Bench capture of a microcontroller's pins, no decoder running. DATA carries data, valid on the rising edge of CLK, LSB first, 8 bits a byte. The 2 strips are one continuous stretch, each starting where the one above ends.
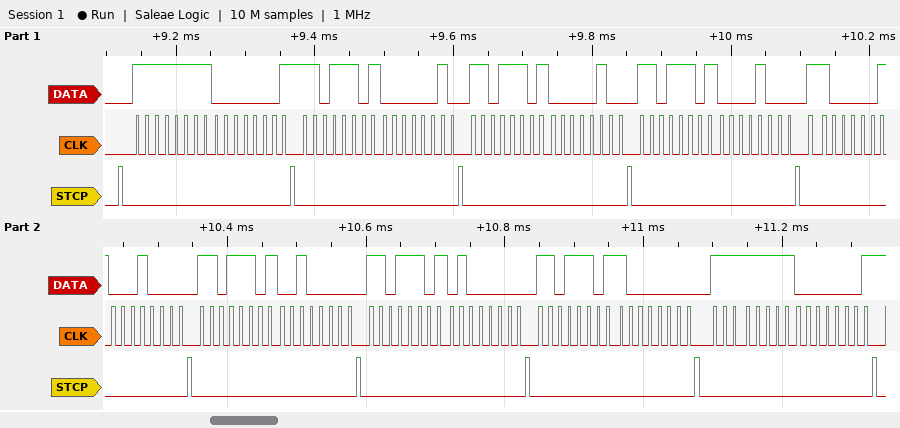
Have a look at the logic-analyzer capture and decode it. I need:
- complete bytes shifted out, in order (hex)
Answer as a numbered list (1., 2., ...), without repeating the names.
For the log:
1. FF 80 BB 40 BB 20 BB 10 83 08 BB 04 BB 02 BB 01 FF 80
